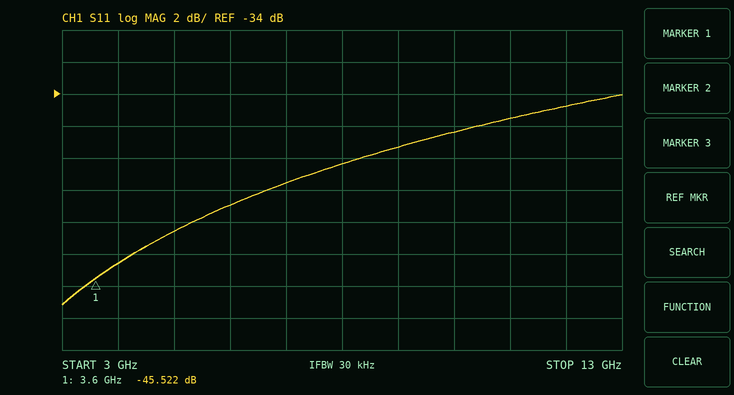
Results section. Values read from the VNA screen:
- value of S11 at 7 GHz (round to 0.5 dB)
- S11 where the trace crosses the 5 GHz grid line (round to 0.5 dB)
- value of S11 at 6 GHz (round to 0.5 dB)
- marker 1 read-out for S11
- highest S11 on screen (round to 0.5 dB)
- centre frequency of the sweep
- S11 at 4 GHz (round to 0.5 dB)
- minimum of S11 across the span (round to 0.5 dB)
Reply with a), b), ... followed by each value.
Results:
a) -39.5 dB
b) -42.5 dB
c) -41.0 dB
d) -45.522 dB
e) -34.0 dB
f) 8 GHz
g) -44.5 dB
h) -47.0 dB
